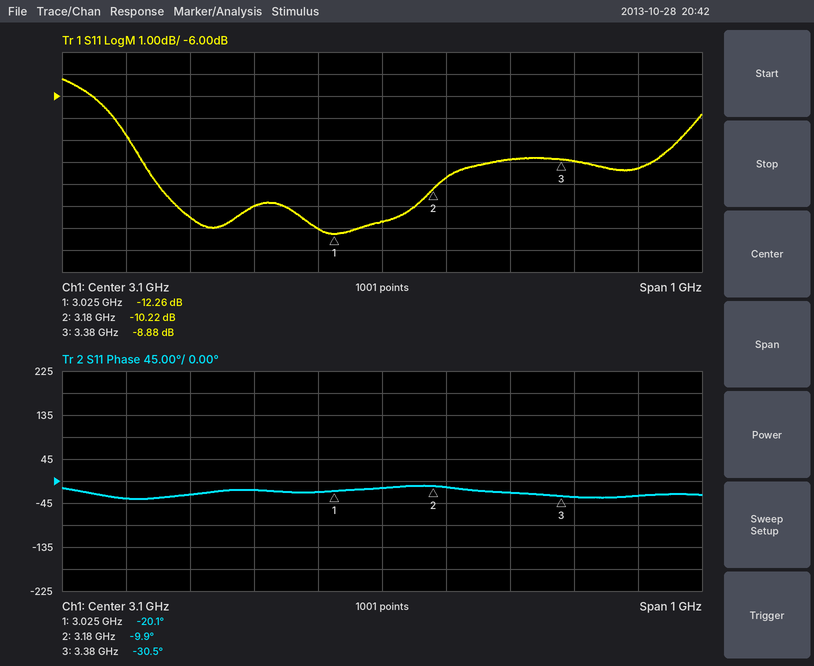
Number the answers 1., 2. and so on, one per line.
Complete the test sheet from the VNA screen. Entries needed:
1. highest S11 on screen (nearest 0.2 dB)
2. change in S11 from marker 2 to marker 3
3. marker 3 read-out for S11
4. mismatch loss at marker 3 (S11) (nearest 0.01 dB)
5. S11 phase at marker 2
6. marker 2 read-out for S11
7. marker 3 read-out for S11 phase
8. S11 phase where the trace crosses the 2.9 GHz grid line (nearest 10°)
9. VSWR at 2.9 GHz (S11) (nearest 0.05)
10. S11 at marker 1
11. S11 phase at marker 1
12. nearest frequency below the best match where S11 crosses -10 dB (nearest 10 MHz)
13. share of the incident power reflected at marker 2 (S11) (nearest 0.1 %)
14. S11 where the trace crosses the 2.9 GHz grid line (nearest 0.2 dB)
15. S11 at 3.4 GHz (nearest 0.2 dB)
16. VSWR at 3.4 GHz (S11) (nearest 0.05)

1. -5.2 dB
2. 1.34 dB
3. -8.88 dB
4. 0.60 dB
5. -9.9°
6. -10.22 dB
7. -30.5°
8. -20°
9. 1.80
10. -12.26 dB
11. -20.1°
12. 2.75 GHz
13. 9.5 %
14. -11.0 dB
15. -9.0 dB
16. 2.10
